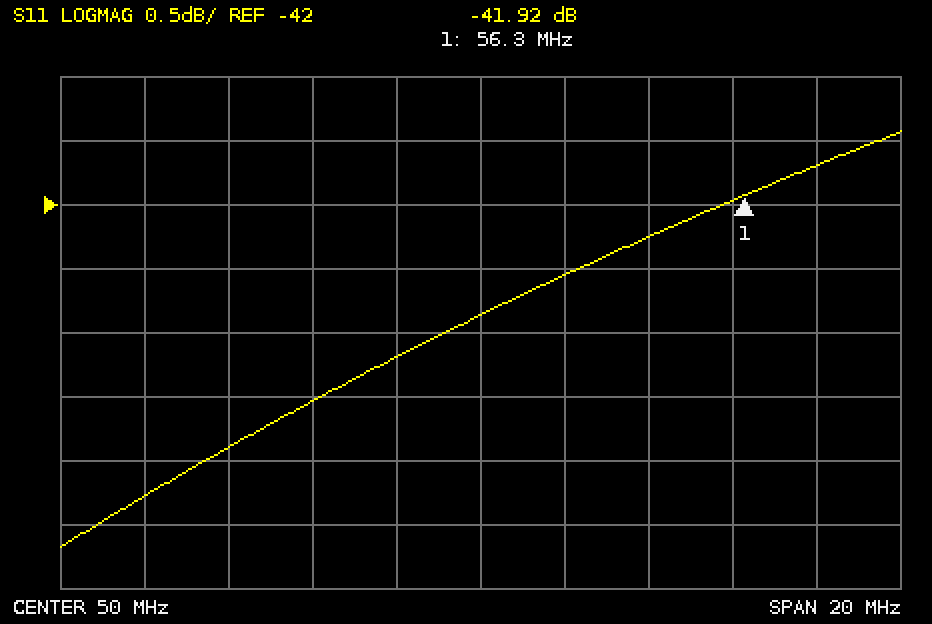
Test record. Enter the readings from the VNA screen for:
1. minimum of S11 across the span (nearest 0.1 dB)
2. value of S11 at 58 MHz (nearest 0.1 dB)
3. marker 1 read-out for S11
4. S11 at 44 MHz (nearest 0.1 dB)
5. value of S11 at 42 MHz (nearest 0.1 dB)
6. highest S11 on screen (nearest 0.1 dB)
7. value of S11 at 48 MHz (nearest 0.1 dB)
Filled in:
-44.7 dB
-41.7 dB
-41.92 dB
-43.9 dB
-44.3 dB
-41.4 dB
-43.2 dB
